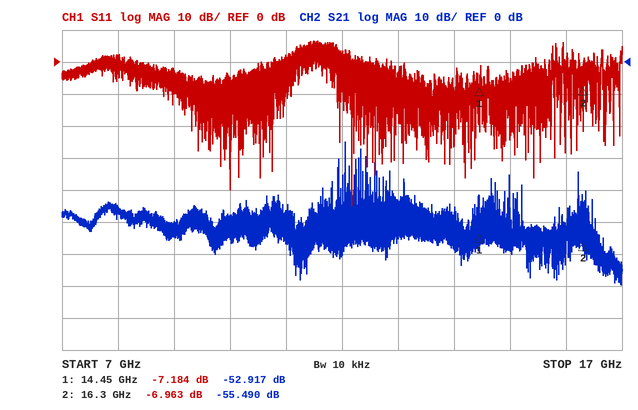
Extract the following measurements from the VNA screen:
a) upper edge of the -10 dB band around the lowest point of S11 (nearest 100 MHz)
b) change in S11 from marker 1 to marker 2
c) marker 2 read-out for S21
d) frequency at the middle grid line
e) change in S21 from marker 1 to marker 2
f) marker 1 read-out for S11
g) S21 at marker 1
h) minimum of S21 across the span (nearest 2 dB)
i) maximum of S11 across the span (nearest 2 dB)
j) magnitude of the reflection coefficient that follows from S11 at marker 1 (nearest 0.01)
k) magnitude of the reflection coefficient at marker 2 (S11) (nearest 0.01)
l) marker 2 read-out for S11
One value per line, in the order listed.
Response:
12.2 GHz
0.221 dB
-55.490 dB
12 GHz
-2.573 dB
-7.184 dB
-52.917 dB
-70 dB
6 dB
0.44
0.45
-6.963 dB
